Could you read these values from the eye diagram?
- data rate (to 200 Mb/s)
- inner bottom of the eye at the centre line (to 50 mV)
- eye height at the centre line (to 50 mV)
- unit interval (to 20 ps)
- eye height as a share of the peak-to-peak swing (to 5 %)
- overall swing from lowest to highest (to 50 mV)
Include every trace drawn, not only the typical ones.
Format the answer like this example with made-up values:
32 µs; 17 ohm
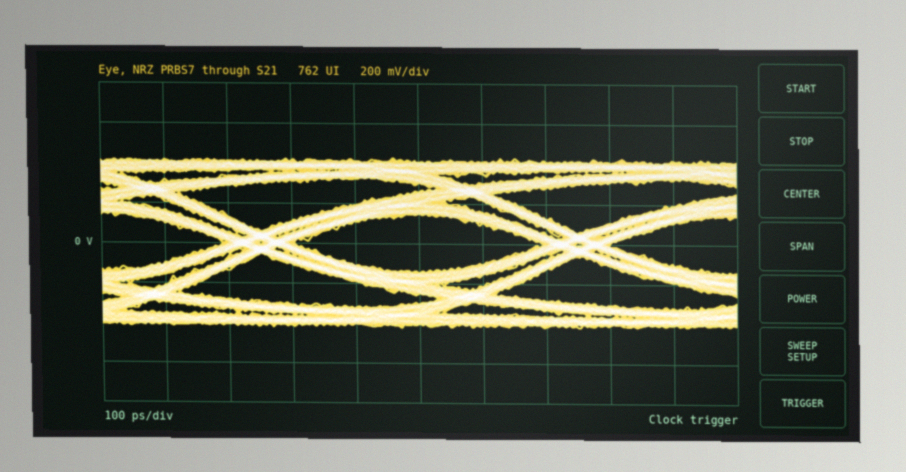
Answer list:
2.0 Gb/s; -150 mV; 300 mV; 500 ps; 35 %; 850 mV
